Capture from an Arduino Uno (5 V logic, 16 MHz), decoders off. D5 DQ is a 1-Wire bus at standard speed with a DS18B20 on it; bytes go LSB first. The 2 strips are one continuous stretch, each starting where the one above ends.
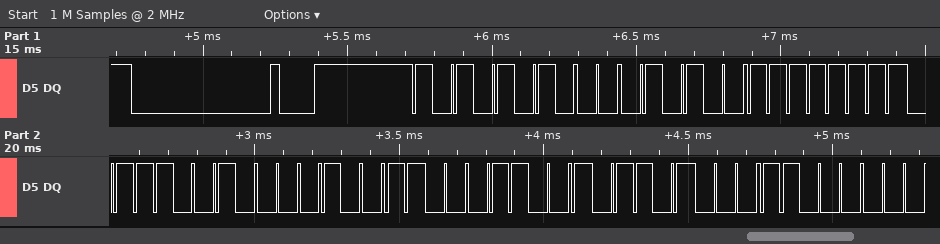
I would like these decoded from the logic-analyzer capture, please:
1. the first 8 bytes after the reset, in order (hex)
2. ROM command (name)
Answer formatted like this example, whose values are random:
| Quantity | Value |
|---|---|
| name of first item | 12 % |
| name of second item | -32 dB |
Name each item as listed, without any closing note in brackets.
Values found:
| Quantity | Value |
|---|---|
| the first 8 bytes after the reset, in order | 55 28 FF 4E C8 98 16 03 |
| ROM command | Match ROM |
